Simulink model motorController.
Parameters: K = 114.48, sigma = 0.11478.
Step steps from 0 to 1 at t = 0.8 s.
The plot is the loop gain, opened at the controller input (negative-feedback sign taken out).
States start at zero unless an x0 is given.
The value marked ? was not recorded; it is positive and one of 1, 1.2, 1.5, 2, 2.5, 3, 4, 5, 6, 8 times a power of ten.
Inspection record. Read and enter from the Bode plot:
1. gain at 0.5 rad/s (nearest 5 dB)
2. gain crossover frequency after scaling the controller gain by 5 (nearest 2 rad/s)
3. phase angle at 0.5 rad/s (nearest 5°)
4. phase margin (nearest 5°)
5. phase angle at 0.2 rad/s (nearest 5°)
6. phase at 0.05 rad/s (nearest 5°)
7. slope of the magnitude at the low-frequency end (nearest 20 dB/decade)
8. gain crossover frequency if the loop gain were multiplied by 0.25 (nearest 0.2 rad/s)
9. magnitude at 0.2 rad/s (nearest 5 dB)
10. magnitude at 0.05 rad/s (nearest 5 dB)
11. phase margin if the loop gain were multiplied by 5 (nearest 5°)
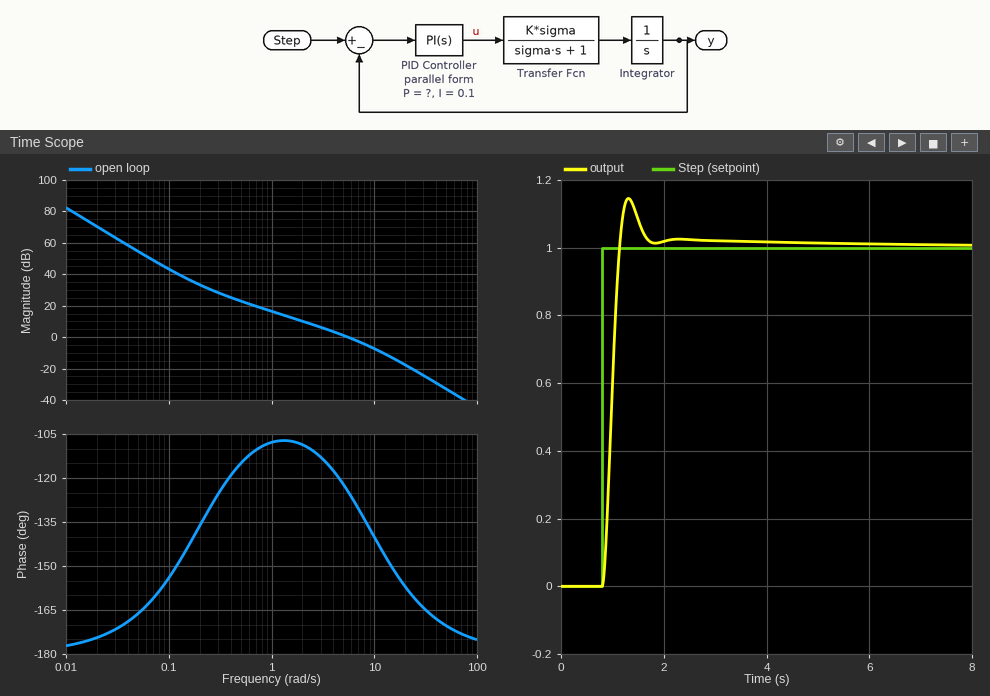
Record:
25 dB
16 rad/s
-115°
55°
-135°
-165°
-40 dB/decade
1.6 rad/s
35 dB
55 dB
30°
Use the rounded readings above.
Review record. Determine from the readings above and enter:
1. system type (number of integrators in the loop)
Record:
2
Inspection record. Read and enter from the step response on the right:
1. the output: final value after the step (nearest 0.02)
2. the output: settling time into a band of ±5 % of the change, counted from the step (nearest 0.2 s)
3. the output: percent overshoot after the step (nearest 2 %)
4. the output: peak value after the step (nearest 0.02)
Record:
1.00
0.8 s
14 %
1.14
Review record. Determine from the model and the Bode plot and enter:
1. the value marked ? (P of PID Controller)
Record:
0.5
